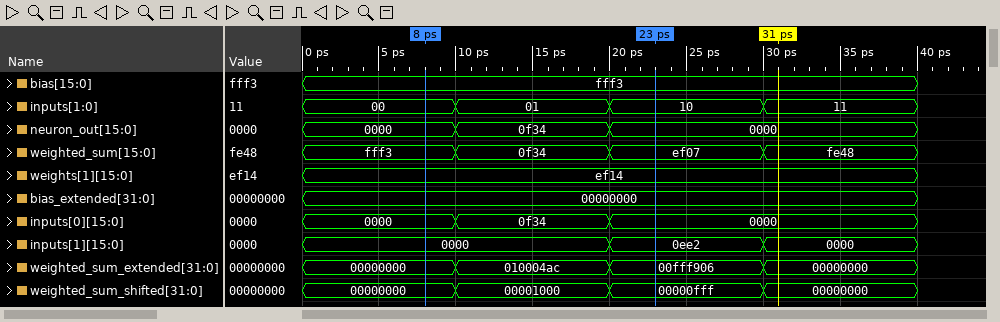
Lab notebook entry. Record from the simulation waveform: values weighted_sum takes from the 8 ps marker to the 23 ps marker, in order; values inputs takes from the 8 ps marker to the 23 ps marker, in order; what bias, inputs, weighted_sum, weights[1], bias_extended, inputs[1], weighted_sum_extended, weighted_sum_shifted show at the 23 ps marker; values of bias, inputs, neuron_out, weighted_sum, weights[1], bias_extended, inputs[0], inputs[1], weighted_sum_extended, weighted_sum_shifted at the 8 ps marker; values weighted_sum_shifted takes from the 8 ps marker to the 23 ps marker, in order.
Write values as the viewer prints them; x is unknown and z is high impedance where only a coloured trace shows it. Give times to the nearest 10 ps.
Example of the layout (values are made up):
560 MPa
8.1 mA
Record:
fff3, 0f34, ef07
00, 01, 10
bias=fff3, inputs=10, weighted_sum=ef07, weights[1]=ef14, bias_extended=00000000, inputs[1]=0ee2, weighted_sum_extended=00fff906, weighted_sum_shifted=00000fff
bias=fff3, inputs=00, neuron_out=0000, weighted_sum=fff3, weights[1]=ef14, bias_extended=00000000, inputs[0]=0000, inputs[1]=0000, weighted_sum_extended=00000000, weighted_sum_shifted=00000000
00000000, 00001000, 00000fff
